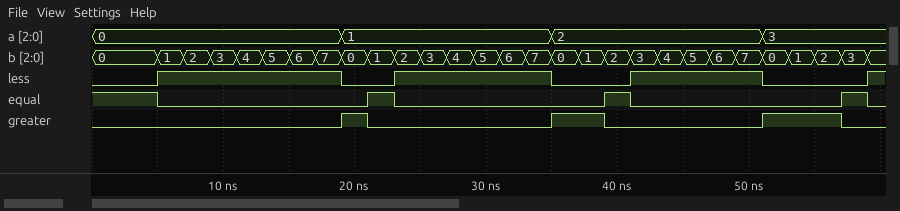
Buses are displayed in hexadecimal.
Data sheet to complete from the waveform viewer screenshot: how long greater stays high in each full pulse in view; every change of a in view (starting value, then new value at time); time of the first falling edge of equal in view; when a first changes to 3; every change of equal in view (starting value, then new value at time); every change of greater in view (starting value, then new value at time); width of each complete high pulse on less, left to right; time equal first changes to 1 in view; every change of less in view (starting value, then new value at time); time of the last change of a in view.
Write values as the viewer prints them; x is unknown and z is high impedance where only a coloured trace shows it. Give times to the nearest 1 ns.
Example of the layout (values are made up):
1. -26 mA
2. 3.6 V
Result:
1. 2 ns, 4 ns, 6 ns
2. 0, 1 at 19 ns, 2 at 35 ns, 3 at 51 ns
3. 5 ns
4. 51 ns
5. 1, 0 at 5 ns, 1 at 21 ns, 0 at 23 ns, 1 at 39 ns, 0 at 41 ns, 1 at 57 ns, 0 at 59 ns
6. 0, 1 at 19 ns, 0 at 21 ns, 1 at 35 ns, 0 at 39 ns, 1 at 51 ns, 0 at 57 ns
7. 14 ns, 12 ns, 10 ns
8. 21 ns
9. 0, 1 at 5 ns, 0 at 19 ns, 1 at 23 ns, 0 at 35 ns, 1 at 41 ns, 0 at 51 ns, 1 at 59 ns
10. 51 ns
